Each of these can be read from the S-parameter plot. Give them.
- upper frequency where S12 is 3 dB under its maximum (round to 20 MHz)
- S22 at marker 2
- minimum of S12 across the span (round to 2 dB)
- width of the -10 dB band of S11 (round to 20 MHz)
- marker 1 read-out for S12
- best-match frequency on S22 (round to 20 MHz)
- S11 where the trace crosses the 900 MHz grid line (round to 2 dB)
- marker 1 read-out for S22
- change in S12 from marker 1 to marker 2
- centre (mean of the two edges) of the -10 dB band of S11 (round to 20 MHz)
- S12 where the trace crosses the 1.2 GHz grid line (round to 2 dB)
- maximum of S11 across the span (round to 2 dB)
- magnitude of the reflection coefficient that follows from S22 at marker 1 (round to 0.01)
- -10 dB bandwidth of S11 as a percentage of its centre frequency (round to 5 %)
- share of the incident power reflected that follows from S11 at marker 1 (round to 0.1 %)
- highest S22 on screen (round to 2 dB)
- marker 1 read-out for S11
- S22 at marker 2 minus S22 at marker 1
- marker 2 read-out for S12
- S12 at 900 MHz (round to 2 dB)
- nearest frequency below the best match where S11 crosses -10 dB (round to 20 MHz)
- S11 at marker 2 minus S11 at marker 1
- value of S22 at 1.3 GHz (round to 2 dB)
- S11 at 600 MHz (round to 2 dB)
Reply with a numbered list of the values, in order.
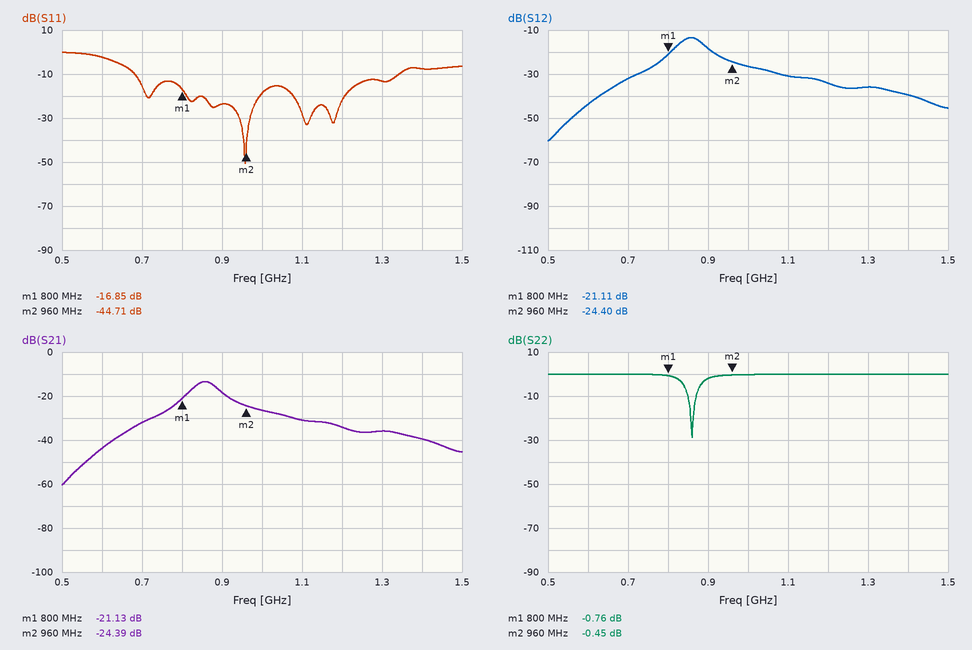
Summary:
1. 880 MHz
2. -0.45 dB
3. -60 dB
4. 660 MHz
5. -21.11 dB
6. 860 MHz
7. -24 dB
8. -0.76 dB
9. -3.29 dB
10. 1.02 GHz
11. -34 dB
12. 0 dB
13. 0.92
14. 65 %
15. 2.1 %
16. 0 dB
17. -16.85 dB
18. 0.31 dB
19. -24.40 dB
20. -18 dB
21. 680 MHz
22. -27.86 dB
23. 0 dB
24. -2 dB
